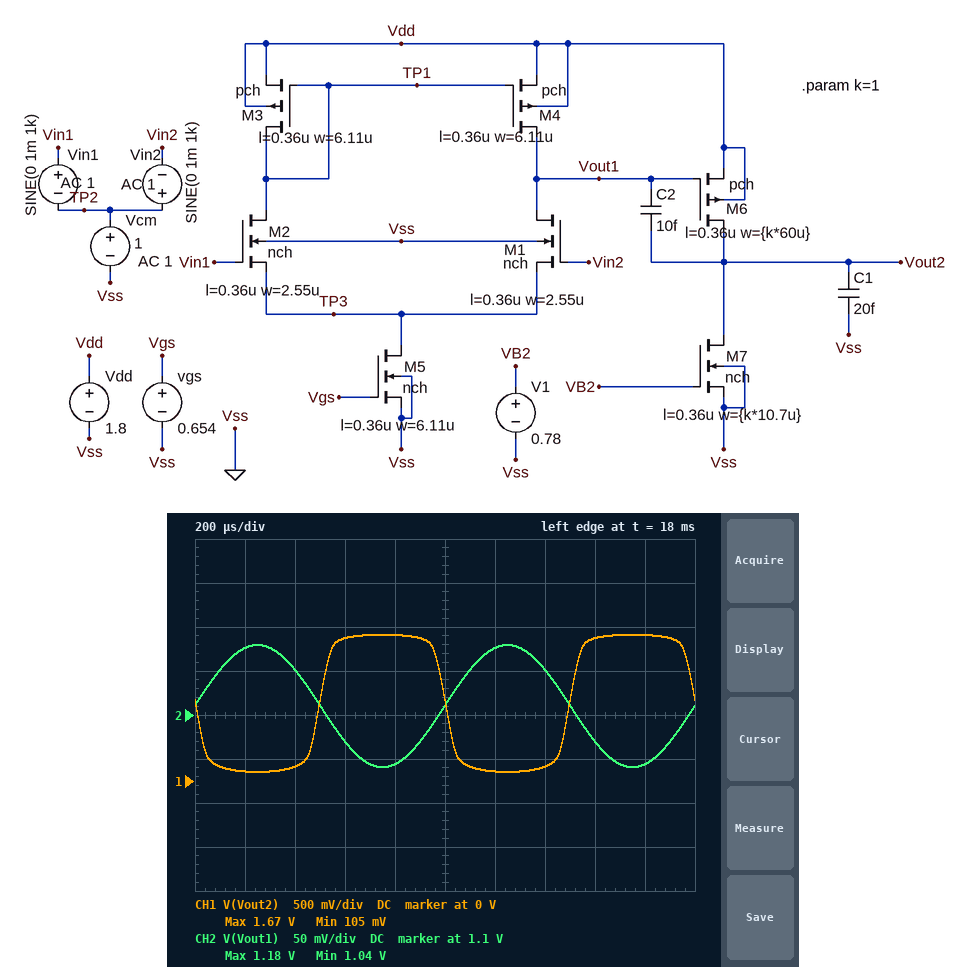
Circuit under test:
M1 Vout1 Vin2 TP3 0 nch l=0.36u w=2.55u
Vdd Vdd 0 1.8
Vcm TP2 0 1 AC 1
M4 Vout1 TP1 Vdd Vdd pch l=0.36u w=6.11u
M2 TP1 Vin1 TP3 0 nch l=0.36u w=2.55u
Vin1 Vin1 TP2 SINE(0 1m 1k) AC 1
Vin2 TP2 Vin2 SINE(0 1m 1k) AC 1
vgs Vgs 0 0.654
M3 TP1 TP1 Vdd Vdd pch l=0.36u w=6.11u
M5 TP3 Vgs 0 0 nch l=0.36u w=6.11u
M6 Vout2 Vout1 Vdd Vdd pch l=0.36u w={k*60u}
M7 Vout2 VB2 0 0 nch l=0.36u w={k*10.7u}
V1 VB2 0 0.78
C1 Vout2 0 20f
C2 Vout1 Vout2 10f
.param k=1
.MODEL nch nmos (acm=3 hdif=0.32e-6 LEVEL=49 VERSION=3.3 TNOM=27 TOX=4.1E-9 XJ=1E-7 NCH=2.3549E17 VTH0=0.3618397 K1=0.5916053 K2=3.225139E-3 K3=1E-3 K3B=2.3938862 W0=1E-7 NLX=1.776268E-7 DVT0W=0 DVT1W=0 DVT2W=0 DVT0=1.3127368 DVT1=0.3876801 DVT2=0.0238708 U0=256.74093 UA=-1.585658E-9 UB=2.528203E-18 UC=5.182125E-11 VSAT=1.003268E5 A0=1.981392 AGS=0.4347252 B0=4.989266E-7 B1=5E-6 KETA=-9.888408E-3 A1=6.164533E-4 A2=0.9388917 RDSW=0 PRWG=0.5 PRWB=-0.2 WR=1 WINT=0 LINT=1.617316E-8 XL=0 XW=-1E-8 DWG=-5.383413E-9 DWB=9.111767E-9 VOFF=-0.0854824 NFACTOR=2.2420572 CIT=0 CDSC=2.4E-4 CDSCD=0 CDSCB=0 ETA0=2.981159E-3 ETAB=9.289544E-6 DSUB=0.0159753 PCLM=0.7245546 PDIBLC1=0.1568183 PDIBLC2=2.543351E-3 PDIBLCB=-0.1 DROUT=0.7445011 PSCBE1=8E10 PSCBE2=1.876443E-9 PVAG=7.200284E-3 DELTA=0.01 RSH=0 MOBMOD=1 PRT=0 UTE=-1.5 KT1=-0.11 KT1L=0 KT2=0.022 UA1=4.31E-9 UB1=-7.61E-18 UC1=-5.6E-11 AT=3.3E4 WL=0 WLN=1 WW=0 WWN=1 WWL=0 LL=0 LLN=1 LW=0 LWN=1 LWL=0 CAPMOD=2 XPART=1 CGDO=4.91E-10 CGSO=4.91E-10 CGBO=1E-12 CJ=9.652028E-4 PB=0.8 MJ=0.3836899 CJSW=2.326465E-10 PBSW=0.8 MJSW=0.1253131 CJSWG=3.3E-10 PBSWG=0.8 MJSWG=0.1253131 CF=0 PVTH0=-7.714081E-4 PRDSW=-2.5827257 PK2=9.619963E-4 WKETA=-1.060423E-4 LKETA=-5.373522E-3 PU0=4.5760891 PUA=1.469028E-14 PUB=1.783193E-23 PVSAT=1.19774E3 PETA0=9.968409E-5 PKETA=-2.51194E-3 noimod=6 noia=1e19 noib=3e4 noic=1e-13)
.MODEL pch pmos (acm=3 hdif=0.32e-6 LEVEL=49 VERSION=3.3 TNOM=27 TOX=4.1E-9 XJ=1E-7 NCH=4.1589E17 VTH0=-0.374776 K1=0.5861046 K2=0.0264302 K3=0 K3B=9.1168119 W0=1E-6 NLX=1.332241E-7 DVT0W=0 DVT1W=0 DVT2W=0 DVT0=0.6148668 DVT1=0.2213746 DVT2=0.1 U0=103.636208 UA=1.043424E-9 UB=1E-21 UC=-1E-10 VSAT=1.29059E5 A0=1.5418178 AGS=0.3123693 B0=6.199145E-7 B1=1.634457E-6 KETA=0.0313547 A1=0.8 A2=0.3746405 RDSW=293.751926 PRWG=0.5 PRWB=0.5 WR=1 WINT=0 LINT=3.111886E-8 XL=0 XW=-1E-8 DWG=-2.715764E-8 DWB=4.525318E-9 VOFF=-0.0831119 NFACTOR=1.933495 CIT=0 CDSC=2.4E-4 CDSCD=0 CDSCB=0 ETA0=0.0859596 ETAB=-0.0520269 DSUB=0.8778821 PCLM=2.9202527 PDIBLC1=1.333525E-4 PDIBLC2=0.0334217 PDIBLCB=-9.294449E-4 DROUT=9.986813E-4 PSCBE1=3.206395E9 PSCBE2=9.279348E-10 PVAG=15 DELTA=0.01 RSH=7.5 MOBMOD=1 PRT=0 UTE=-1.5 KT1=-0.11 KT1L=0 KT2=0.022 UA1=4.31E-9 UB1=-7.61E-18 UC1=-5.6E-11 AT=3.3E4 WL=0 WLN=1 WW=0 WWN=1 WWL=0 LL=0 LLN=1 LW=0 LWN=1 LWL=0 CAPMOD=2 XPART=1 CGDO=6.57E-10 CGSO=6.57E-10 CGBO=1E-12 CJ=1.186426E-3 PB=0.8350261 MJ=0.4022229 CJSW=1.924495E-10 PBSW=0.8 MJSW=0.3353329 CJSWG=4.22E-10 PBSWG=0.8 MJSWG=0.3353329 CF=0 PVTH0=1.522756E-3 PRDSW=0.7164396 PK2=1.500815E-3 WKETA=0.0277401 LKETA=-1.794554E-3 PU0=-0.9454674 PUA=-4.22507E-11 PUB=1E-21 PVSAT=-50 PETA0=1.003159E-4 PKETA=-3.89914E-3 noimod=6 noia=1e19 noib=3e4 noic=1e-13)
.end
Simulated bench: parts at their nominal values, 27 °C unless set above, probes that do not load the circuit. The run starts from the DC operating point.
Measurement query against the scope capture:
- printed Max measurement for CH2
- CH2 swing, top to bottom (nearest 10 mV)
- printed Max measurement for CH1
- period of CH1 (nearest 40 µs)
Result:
1.18 V
140 mV
1.67 V
1.00 ms
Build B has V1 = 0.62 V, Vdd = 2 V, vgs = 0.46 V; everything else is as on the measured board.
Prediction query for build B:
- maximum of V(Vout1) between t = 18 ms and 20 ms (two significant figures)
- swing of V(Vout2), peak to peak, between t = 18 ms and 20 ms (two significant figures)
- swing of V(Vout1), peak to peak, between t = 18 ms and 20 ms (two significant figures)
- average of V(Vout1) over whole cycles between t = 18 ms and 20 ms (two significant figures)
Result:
1.6 V
150 mV
160 mV
1.5 V
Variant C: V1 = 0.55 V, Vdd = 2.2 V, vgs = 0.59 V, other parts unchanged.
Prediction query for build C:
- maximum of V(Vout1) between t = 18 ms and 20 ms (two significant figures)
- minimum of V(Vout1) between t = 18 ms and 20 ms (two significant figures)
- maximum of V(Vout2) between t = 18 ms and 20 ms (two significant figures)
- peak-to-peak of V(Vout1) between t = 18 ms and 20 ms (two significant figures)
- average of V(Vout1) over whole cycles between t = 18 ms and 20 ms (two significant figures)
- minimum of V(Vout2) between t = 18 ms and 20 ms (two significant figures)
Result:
1.7 V
1.5 V
2.2 V
160 mV
1.6 V
2.1 V
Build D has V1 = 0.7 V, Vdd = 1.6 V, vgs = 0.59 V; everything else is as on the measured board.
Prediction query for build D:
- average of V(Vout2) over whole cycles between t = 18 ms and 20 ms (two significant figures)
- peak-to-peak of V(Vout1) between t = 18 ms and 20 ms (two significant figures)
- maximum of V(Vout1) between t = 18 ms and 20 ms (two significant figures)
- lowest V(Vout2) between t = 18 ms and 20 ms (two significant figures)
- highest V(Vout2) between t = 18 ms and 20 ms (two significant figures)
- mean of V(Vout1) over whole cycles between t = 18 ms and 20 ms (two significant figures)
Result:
660 mV
150 mV
1.1 V
38 mV
1.5 V
990 mV
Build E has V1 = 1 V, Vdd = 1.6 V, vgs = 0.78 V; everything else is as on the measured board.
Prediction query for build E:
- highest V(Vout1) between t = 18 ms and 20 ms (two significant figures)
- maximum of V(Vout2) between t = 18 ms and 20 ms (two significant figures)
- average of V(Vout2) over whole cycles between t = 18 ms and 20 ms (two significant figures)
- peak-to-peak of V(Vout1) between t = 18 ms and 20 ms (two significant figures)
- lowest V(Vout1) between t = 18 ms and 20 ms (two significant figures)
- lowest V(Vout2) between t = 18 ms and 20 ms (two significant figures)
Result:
820 mV
1.3 V
620 mV
100 mV
720 mV
210 mV
